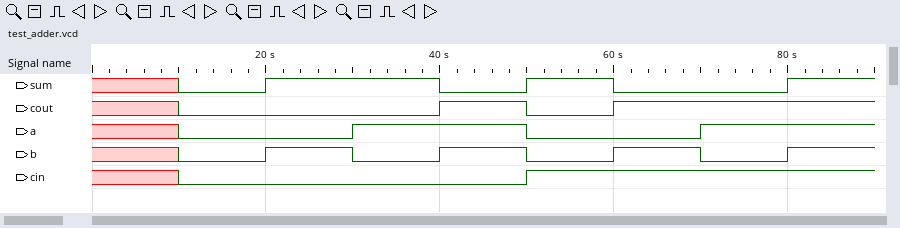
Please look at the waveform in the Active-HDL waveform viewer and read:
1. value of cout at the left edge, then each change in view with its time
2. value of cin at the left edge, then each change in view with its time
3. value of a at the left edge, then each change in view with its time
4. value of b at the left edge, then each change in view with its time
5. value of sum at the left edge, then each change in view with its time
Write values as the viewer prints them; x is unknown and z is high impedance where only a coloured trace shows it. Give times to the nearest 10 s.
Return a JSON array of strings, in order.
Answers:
["x, 0 at 10 s, 1 at 40 s, 0 at 50 s, 1 at 60 s", "x, 0 at 10 s, 1 at 50 s", "x, 0 at 10 s, 1 at 30 s, 0 at 50 s, 1 at 70 s", "x, 0 at 10 s, 1 at 20 s, 0 at 30 s, 1 at 40 s, 0 at 50 s, 1 at 60 s, 0 at 70 s, 1 at 80 s", "x, 0 at 10 s, 1 at 20 s, 0 at 40 s, 1 at 50 s, 0 at 60 s, 1 at 80 s"]
